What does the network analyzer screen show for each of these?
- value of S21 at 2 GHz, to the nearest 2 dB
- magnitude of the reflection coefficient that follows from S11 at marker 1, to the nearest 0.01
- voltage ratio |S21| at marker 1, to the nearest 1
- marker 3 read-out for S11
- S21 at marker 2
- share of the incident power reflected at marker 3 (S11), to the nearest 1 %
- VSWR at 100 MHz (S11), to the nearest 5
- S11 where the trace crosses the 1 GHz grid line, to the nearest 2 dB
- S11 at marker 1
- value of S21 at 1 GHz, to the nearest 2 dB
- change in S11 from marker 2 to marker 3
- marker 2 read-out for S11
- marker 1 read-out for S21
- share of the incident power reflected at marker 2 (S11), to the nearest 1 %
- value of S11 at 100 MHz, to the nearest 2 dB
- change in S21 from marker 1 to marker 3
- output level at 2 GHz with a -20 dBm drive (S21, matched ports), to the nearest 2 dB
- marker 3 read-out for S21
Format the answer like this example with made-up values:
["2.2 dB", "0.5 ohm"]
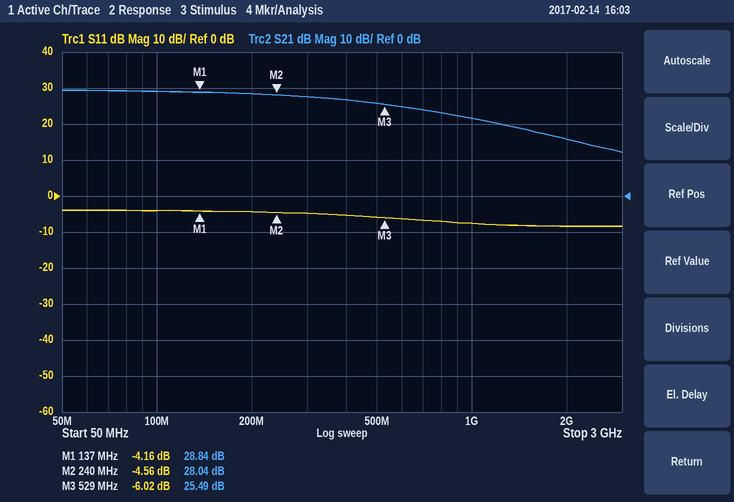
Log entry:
["16 dB", "0.62", "28", "-6.02 dB", "28.04 dB", "25 %", "5", "-8 dB", "-4.16 dB", "22 dB", "-1.46 dB", "-4.56 dB", "28.84 dB", "35 %", "-4 dB", "-3.35 dB", "-4 dBm", "25.49 dB"]
